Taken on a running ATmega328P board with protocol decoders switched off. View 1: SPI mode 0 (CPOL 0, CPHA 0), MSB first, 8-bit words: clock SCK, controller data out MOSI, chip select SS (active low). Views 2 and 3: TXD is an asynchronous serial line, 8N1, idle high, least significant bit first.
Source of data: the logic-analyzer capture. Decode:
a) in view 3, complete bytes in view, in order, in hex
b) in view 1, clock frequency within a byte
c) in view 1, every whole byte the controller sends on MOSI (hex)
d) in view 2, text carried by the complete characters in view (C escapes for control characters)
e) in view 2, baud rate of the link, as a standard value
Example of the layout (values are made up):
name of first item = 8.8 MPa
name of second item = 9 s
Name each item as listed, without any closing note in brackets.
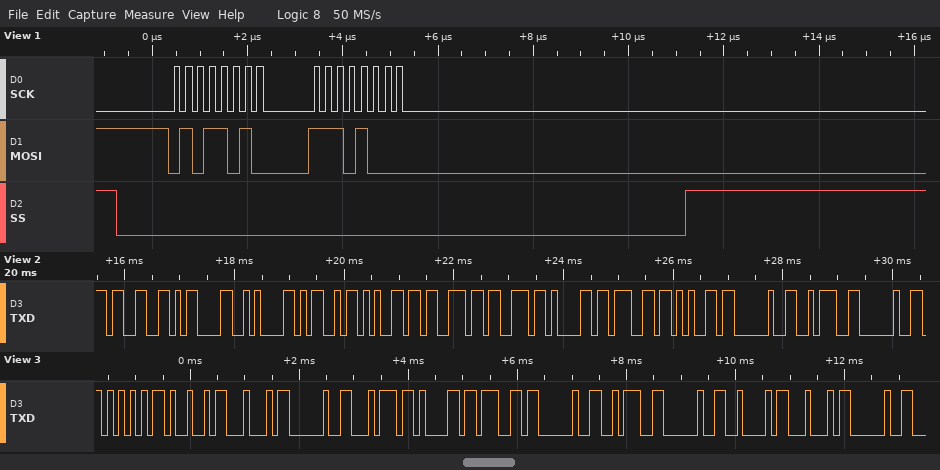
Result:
in view 3, complete bytes in view, in order, in hex = 0x55 0x49 0x44 0x20 0x74 0x61 0x67 0x20 0x3A 0x20 0x42 0x44 0x20
in view 1, clock frequency within a byte = 4 MHz
in view 1, every whole byte the controller sends on MOSI = 5A E8
in view 2, text carried by the complete characters in view = "3\r\nMessage : "
in view 2, baud rate of the link, as a standard value = 9600 baud
